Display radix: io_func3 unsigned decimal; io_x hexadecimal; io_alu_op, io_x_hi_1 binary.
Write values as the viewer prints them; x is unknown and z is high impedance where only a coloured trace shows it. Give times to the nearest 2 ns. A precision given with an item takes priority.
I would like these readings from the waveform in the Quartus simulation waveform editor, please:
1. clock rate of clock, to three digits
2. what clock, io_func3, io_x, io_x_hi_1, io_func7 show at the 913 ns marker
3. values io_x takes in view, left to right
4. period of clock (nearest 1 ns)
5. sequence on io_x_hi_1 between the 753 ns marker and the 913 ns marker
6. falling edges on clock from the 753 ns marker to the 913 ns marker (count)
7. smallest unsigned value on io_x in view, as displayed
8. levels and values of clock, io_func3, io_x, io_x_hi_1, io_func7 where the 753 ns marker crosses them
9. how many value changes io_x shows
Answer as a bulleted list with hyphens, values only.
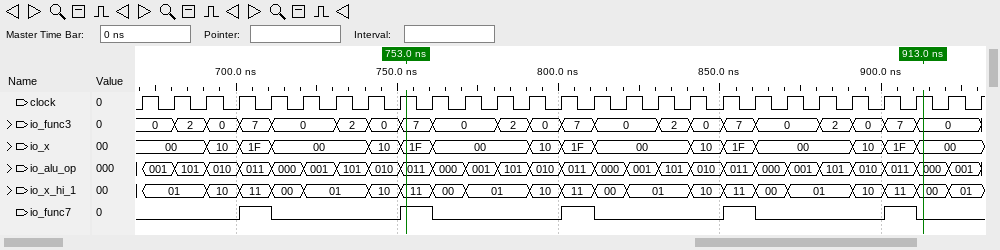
- 100 MHz
- clock=1, io_func3=0, io_x=00, io_x_hi_1=00, io_func7=0
- 00, 10, 1F, 00, 10, 1F, 00, 10, 1F, 00, 10, 1F, 00, 10, 1F, 00
- 10 ns
- 11, 00, 01, 10, 11, 00, 01, 10, 11, 00, 01, 10, 11, 00
- 16
- 00
- clock=1, io_func3=7, io_x=1F, io_x_hi_1=11, io_func7=1
- 15
